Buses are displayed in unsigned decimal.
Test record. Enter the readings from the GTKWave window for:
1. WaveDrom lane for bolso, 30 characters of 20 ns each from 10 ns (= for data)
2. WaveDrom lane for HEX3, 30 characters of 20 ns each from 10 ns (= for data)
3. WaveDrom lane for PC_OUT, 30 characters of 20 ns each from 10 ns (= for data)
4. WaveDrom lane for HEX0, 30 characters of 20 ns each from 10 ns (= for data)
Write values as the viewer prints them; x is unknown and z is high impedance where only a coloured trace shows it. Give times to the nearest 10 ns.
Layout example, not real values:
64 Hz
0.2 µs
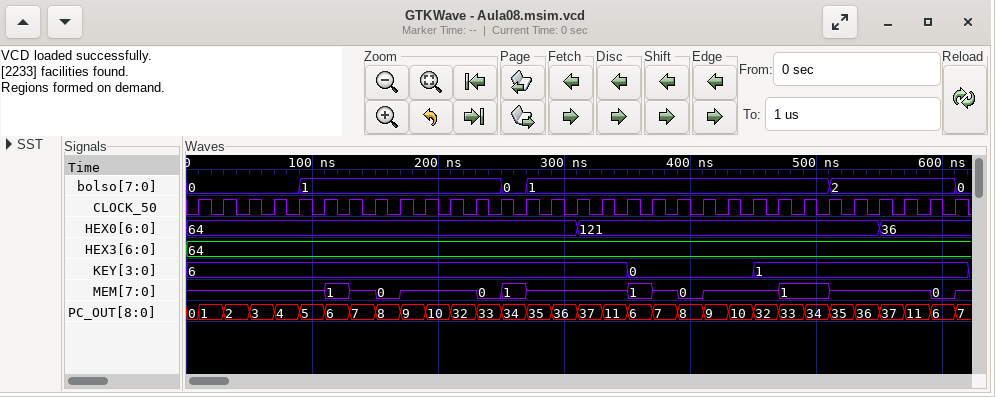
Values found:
{name: 'bolso', wave: '=...=.......==...........=....', data: '0 1 0 1 2'}
{name: 'HEX3', wave: '=.............................', data: '64'}
{name: 'PC_OUT', wave: '==============================', data: '1 2 3 4 5 6 7 8 9 10 32 33 34 35 36 37 11 6 7 8 9 10 32 33 34 35 36 37 11 6'}
{name: 'HEX0', wave: '=..............=...........=..', data: '64 121 36'}
